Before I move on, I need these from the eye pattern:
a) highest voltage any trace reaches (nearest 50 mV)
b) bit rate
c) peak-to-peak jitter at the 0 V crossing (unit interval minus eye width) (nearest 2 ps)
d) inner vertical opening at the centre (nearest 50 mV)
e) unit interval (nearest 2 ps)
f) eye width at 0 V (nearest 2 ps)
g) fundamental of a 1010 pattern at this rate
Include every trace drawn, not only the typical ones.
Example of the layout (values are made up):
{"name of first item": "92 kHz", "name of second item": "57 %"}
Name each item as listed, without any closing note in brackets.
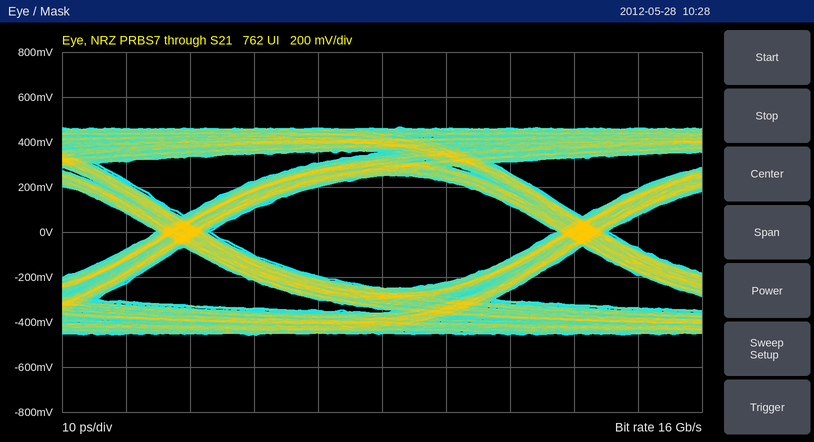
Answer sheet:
{"highest voltage any trace reaches": "450 mV", "bit rate": "16 Gb/s", "peak-to-peak jitter at the 0 V crossing (unit interval minus eye width)": "8 ps", "inner vertical opening at the centre": "500 mV", "unit interval": "62 ps", "eye width at 0 V": "54 ps", "fundamental of a 1010 pattern at this rate": "8 GHz"}
